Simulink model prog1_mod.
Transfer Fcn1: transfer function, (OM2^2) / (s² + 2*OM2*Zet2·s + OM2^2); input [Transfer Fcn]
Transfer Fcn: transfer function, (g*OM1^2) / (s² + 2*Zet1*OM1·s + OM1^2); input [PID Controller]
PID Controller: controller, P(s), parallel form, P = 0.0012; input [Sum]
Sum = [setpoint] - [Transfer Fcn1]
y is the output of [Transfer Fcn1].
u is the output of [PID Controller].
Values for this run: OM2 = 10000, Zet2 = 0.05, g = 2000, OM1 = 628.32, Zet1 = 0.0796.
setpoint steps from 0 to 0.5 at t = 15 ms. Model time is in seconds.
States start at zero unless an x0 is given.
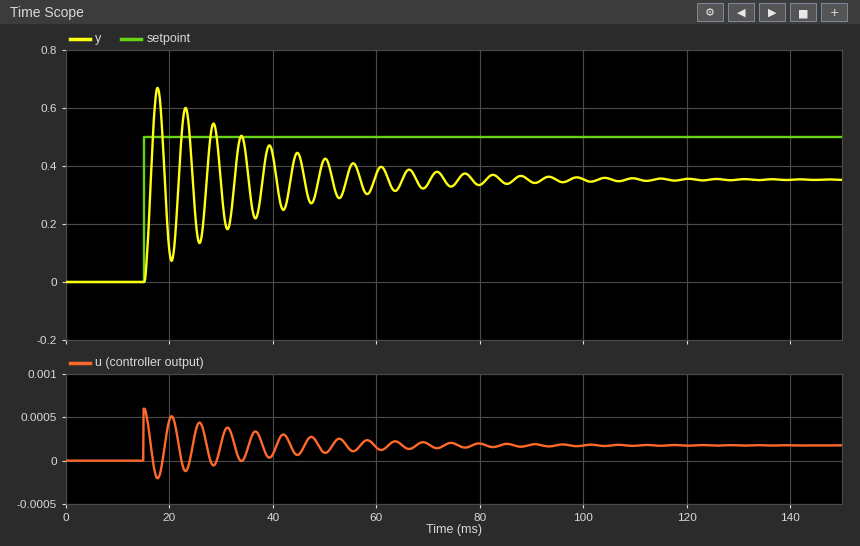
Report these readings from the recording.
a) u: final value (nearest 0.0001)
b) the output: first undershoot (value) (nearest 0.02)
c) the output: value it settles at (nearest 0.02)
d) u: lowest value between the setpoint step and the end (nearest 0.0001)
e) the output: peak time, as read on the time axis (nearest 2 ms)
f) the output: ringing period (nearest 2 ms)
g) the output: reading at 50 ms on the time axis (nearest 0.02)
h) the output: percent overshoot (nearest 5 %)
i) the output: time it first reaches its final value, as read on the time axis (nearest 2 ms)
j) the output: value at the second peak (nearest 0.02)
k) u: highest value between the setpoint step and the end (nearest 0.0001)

0.0002
0.08
0.36
-0.0002
18 ms
6 ms
0.42
90 %
16 ms
0.60
0.0006
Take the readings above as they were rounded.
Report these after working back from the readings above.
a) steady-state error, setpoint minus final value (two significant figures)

0.14
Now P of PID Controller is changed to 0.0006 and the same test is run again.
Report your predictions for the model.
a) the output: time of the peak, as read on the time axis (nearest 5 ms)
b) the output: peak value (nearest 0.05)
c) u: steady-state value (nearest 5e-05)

20 ms
0.50
0.00015
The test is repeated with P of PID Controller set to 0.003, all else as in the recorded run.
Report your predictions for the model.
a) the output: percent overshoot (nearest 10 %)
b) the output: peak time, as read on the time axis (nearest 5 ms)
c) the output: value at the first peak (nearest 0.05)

100 %
15 ms
0.85
